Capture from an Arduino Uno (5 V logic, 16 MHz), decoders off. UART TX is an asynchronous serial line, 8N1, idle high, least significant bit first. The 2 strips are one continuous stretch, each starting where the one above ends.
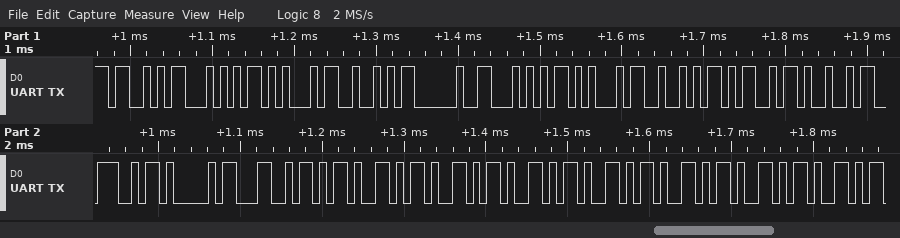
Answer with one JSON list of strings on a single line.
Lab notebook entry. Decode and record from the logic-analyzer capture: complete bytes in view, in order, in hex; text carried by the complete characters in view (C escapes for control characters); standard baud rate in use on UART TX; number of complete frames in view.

["53 54 45 52 20 54 45 52 4D 49 4E 41 4C 2D 2D 2D 2D 2D 2D 2D", "\"STER TERMINAL-------\"", "115200 baud", "20"]
